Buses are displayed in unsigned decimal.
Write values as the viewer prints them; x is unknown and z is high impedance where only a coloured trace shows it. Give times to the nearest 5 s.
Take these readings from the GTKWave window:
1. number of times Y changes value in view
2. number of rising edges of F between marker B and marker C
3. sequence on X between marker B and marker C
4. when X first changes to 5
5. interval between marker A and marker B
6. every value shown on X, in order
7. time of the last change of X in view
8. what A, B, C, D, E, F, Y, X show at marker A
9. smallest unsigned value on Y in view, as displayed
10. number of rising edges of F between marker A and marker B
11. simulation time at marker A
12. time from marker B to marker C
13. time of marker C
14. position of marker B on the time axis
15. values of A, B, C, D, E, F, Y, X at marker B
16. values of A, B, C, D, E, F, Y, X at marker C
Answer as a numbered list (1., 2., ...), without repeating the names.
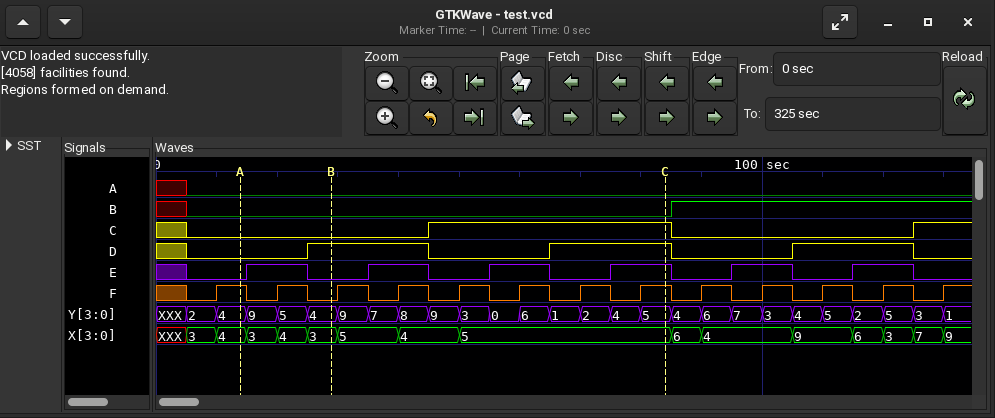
1. 26
2. 6
3. 3, 5, 4, 5
4. 30 s
5. 15 s
6. XXX, 3, 4, 3, 4, 3, 5, 4, 5, 6, 4, 9, 6, 3, 7, 9
7. 130 s
8. A=0, B=0, C=0, D=0, E=0, F=1, Y=4, X=4
9. 0
10. 1
11. 15 s
12. 55 s
13. 85 s
14. 30 s
15. A=0, B=0, C=0, D=1, E=0, F=0, Y=4, X=3
16. A=0, B=0, C=1, D=1, E=1, F=1, Y=5, X=5
